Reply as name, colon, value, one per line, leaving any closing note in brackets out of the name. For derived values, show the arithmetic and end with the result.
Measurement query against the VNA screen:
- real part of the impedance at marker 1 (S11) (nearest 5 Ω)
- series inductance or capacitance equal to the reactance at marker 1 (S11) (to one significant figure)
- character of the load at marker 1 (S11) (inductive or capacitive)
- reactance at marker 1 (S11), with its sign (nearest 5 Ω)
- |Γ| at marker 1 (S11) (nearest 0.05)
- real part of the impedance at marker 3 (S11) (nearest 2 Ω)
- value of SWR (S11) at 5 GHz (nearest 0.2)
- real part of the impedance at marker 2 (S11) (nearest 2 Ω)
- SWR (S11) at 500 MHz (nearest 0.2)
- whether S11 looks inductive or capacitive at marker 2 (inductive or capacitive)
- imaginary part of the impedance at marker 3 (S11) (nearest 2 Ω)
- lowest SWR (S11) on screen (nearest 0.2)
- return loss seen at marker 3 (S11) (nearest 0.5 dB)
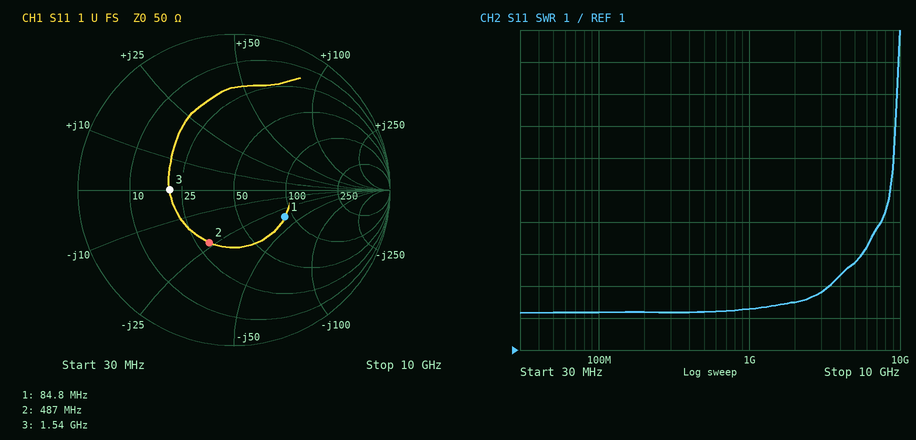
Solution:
real part of the impedance at marker 1 (S11): 90 Ω
series inductance or capacitance equal to the reactance at marker 1 (S11): C = 1/(2π × 84.8 MHz × 35 Ω) ≈ 53.6 pF, so 50 pF to one significant figure
character of the load at marker 1 (S11): capacitive
reactance at marker 1 (S11), with its sign: -35 Ω
|Γ| at marker 1 (S11): 0.35
real part of the impedance at marker 3 (S11): 20 Ω
value of SWR (S11) at 5 GHz: 3.8
real part of the impedance at marker 2 (S11): 30 Ω
SWR (S11) at 500 MHz: 2.2
whether S11 looks inductive or capacitive at marker 2: capacitive
imaginary part of the impedance at marker 3 (S11): 0 Ω
lowest SWR (S11) on screen: 2.2
return loss seen at marker 3 (S11): 7.5 dB
